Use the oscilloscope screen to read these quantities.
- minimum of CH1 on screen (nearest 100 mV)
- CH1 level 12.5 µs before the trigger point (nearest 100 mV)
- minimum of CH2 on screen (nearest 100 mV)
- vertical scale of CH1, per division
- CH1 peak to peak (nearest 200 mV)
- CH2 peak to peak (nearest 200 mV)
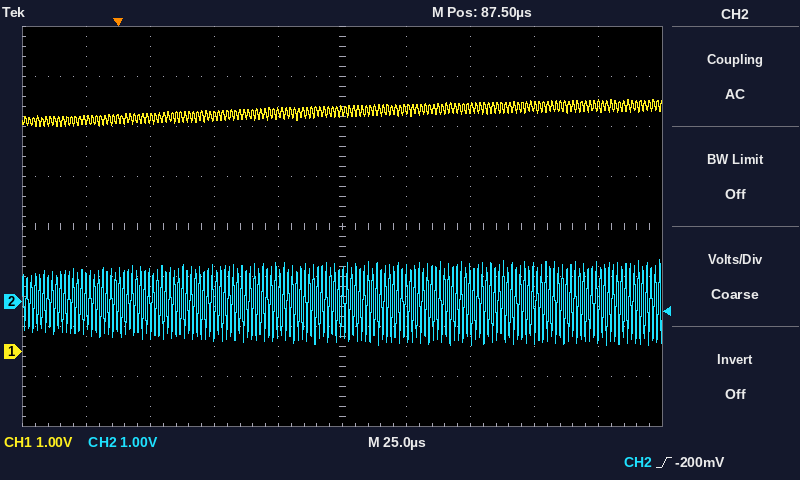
4.5 V
4.6 V
-900 mV
1 V
600 mV
1.8 V
